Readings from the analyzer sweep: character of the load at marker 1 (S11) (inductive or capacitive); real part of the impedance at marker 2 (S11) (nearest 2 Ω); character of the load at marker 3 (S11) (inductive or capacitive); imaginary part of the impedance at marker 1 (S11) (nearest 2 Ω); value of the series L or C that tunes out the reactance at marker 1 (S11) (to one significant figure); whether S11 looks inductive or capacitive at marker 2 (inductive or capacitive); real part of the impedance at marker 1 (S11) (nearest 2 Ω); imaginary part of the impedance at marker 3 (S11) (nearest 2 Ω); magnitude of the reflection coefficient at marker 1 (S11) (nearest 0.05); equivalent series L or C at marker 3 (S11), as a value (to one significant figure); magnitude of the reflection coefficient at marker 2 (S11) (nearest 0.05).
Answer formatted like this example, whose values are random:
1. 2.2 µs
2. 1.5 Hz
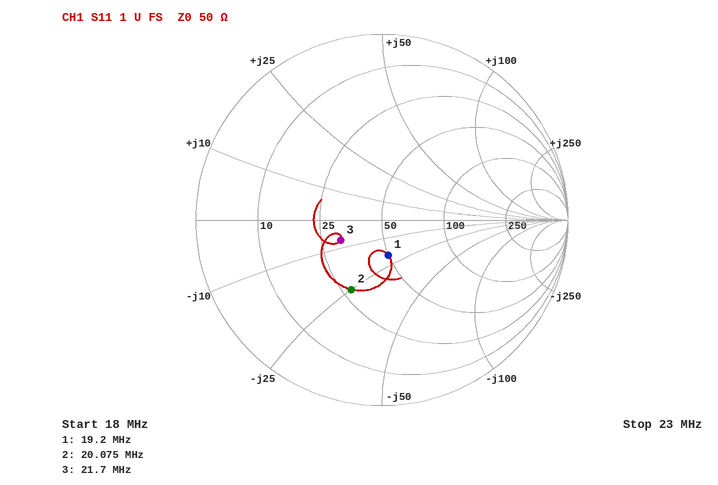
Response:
1. capacitive
2. 28 Ω
3. capacitive
4. -20 Ω
5. 200 nH
6. capacitive
7. 50 Ω
8. -8 Ω
9. 0.20
10. 1 nF
11. 0.40
